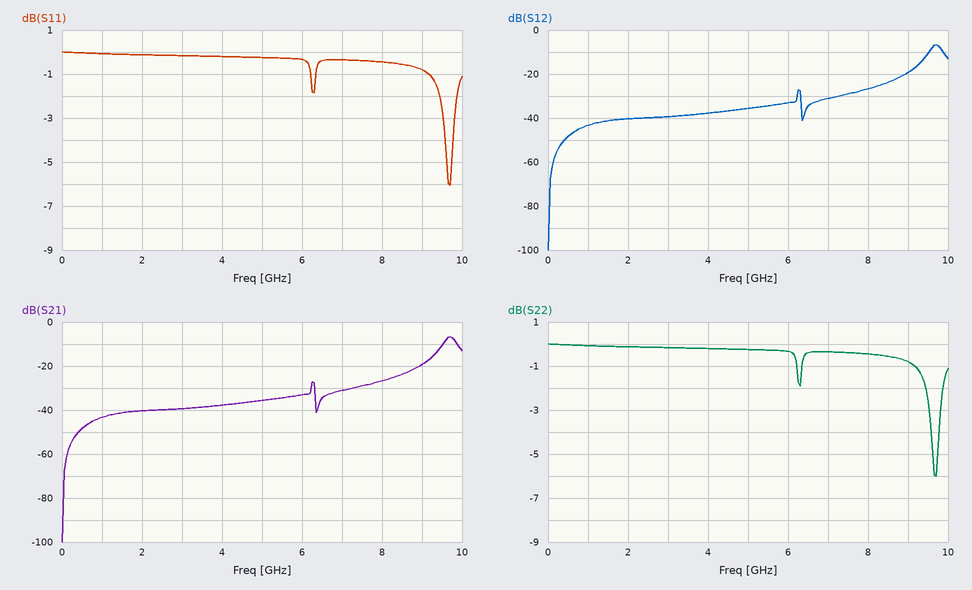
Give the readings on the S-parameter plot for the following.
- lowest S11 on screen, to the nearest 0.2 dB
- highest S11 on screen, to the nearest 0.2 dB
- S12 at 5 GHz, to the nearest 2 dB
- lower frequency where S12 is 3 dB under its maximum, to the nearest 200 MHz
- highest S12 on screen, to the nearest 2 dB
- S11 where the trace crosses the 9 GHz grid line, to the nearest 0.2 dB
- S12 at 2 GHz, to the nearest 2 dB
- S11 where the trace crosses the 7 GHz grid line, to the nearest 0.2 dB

-6.0 dB
0.0 dB
-36 dB
9.6 GHz
-6 dB
-0.8 dB
-40 dB
-0.4 dB
